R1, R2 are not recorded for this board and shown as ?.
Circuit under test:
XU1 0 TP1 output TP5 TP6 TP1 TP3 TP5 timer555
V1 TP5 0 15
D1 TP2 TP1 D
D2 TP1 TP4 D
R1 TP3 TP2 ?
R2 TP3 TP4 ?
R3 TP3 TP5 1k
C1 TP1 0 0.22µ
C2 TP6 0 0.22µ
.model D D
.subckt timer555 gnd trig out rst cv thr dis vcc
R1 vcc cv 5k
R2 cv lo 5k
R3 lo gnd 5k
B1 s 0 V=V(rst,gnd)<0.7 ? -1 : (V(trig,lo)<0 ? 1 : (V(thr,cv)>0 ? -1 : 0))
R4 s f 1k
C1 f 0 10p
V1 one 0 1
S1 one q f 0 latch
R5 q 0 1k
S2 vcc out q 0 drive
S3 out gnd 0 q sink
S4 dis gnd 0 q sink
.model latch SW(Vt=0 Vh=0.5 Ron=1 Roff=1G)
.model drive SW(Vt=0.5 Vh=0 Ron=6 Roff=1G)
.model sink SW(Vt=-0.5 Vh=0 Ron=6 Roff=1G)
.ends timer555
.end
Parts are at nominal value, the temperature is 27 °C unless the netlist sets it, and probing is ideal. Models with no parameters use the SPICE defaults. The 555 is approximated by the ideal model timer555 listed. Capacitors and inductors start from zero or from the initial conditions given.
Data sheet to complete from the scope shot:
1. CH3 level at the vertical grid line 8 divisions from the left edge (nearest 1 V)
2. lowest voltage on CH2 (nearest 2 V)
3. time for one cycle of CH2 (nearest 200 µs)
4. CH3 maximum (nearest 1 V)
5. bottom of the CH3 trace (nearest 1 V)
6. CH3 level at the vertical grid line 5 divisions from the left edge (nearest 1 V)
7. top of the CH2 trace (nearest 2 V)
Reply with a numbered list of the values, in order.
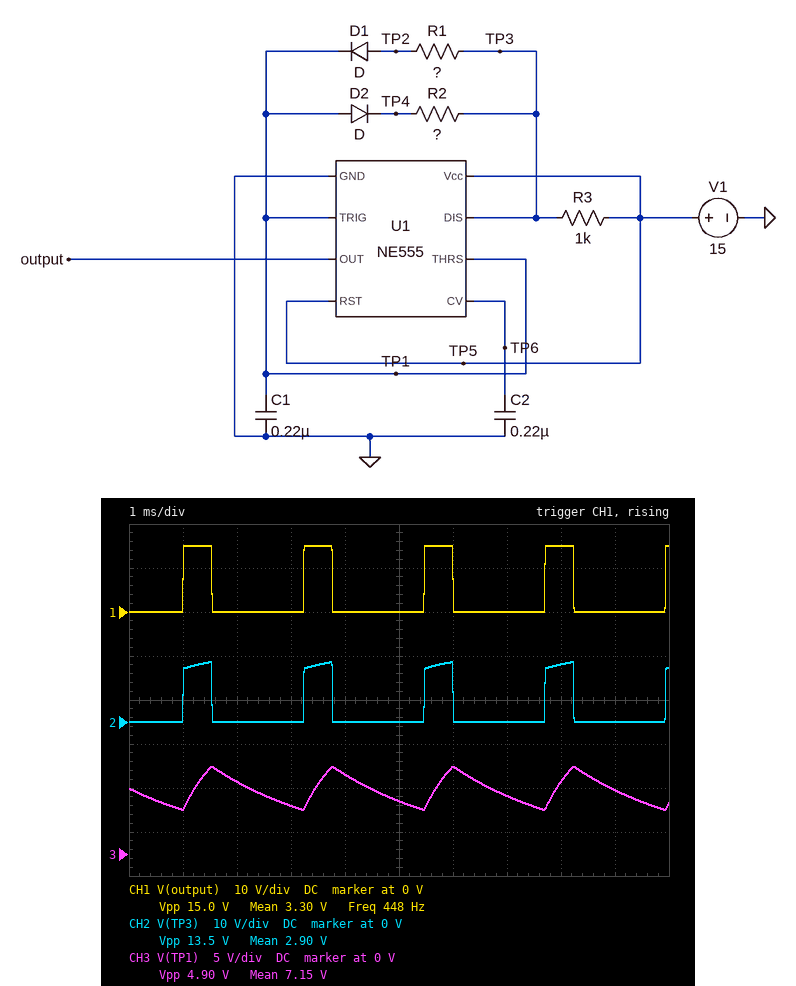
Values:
1. 8 V
2. 0 V
3. 2.2 ms
4. 10 V
5. 5 V
6. 6 V
7. 14 V
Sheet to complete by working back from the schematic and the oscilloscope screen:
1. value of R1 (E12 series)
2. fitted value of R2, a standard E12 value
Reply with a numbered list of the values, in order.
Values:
1. 2.2 kΩ
2. 10 kΩ
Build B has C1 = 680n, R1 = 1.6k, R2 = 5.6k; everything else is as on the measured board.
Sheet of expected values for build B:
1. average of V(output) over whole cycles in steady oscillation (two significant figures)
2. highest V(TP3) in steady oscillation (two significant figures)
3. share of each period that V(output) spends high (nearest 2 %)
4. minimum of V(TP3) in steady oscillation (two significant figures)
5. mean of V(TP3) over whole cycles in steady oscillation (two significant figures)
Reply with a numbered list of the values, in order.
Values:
1. 4.7 V
2. 13 V
3. 32 %
4. 94 mV
5. 4.0 V
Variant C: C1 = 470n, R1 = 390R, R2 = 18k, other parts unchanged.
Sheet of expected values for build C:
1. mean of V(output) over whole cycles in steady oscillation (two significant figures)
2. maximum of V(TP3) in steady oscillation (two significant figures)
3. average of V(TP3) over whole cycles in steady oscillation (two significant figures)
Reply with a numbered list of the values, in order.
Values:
1. 1.1 V
2. 12 V
3. 820 mV
